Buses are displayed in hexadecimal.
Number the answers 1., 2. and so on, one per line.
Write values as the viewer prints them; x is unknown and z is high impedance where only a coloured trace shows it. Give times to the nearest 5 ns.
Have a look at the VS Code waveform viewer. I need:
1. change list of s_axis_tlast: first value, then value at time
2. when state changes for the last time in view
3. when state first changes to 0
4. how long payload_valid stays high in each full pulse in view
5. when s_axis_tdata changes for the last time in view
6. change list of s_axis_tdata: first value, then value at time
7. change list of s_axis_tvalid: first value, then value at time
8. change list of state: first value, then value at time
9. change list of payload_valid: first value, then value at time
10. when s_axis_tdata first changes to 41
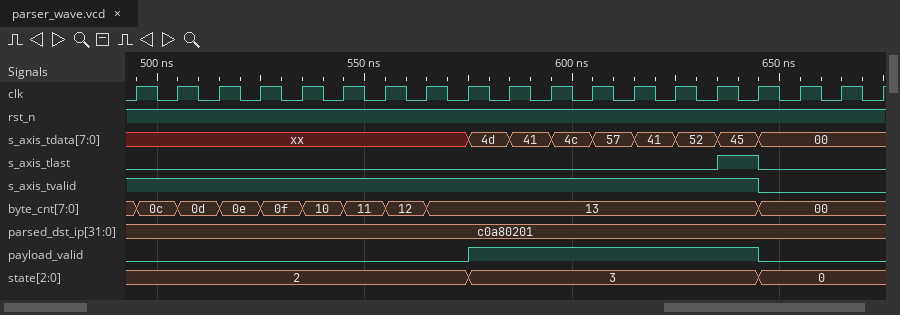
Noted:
1. 0, 1 at 635 ns, 0 at 645 ns
2. 645 ns
3. 645 ns
4. 70 ns
5. 645 ns
6. xx, 4d at 575 ns, 41 at 585 ns, 4c at 595 ns, 57 at 605 ns, 41 at 615 ns, 52 at 625 ns, 45 at 635 ns, 00 at 645 ns
7. 1, 0 at 645 ns
8. 2, 3 at 575 ns, 0 at 645 ns
9. 0, 1 at 575 ns, 0 at 645 ns
10. 585 ns
